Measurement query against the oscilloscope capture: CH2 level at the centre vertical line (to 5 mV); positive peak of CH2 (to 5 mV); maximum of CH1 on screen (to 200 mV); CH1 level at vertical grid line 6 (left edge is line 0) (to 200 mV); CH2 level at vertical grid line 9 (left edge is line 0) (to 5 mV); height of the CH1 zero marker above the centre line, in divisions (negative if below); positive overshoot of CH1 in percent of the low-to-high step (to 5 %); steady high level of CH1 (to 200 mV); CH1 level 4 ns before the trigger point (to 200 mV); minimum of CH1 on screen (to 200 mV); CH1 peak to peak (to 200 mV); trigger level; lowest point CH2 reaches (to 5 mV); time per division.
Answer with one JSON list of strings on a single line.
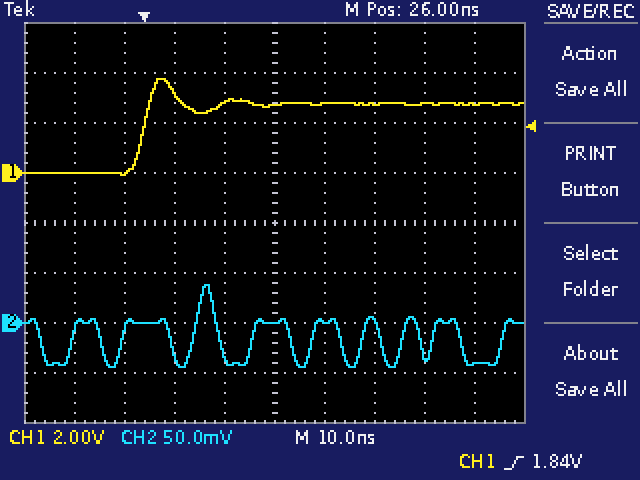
["0 mV", "40 mV", "3.8 V", "2.8 V", "-40 mV", "+1.0 div", "35 %", "2.8 V", "0.0 V", "0.0 V", "3.8 V", "1.84 V", "-45 mV", "10 ns"]
